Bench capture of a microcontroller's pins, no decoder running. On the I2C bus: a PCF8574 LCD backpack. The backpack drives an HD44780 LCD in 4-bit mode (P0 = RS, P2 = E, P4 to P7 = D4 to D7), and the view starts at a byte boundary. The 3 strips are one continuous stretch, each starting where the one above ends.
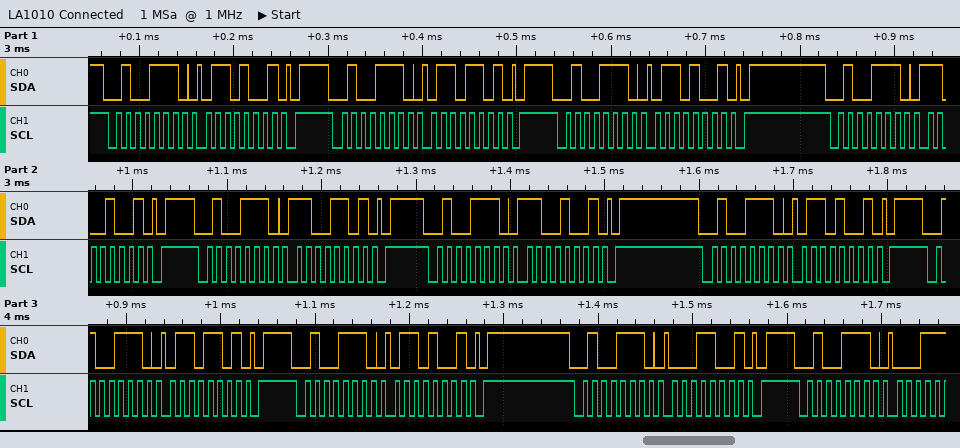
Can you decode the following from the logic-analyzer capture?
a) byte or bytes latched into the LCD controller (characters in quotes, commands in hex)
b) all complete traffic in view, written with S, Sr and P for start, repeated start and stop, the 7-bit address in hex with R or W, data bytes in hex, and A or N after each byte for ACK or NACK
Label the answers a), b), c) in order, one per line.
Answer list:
a) 'l'
b) S 27W A 69 A P S 27W A 6D A P S 27W A 69 A P S 27W A C9 A P S 27W A CD A P S 27W A C9 A P S 27W A 69 A P S 27W A 6D A P S 27W A 69 A P S 27W A 19 A P S 27W A
